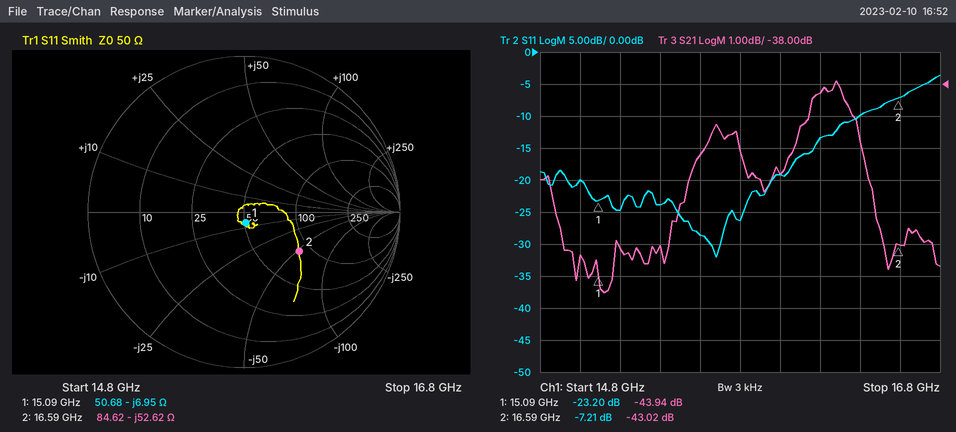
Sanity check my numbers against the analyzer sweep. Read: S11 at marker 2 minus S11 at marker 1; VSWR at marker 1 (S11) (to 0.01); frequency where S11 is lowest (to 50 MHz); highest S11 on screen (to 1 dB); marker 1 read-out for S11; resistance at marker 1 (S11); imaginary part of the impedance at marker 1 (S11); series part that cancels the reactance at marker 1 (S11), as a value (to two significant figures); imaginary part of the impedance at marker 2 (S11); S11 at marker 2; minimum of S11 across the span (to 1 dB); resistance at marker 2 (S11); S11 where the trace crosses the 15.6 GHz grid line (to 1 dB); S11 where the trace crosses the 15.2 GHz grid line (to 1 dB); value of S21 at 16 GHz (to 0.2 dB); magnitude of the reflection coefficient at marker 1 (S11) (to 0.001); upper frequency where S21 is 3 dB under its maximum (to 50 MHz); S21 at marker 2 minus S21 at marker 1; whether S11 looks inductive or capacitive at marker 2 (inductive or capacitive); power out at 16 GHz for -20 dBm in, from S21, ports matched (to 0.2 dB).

15.99 dB
1.15
15.70 GHz
-4 dB
-23.20 dB
50.68 Ω
-6.95 Ω
73 pH
-52.62 Ω
-7.21 dB
-32 dB
84.62 Ω
-29 dB
-25 dB
-40.8 dB
0.069
16.45 GHz
0.92 dB
capacitive
-60.8 dBm
